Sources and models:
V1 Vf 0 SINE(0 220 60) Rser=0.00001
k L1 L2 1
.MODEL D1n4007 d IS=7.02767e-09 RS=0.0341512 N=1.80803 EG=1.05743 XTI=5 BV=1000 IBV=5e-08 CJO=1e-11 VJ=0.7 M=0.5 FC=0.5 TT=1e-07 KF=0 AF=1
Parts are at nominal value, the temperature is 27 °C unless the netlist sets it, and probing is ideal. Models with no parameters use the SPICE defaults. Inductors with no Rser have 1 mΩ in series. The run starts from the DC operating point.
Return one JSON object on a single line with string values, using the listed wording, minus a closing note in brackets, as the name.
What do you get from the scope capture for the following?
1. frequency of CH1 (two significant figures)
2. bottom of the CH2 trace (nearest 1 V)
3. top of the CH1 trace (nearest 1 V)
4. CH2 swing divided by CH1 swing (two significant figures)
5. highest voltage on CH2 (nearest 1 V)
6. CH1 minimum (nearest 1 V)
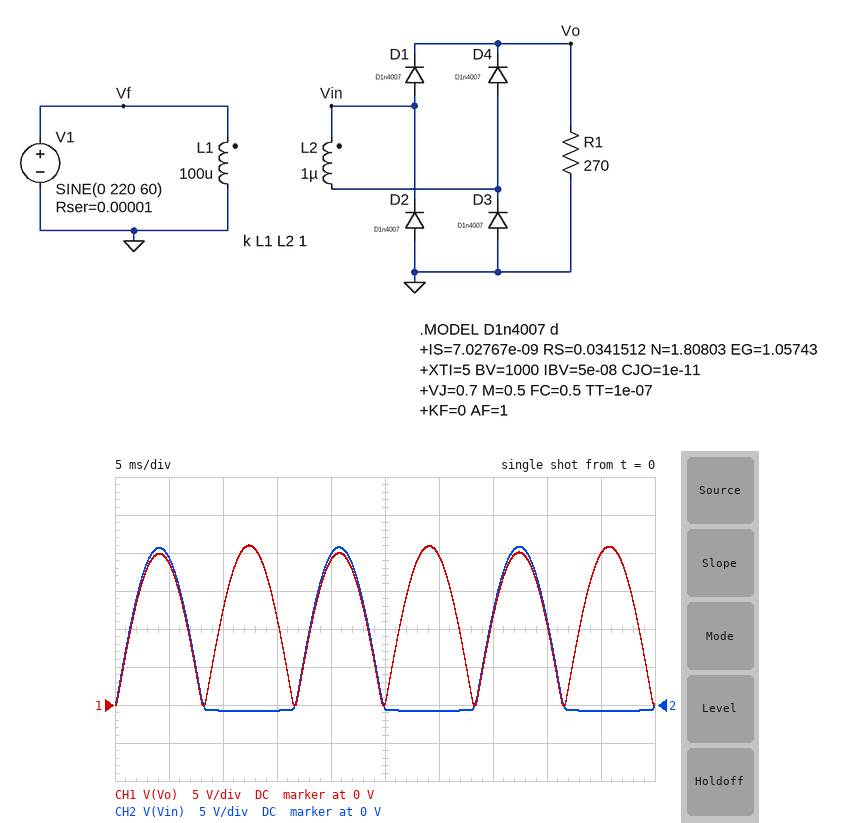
{"frequency of CH1": "120 Hz", "bottom of the CH2 trace": "-1 V", "top of the CH1 trace": "21 V", "CH2 swing divided by CH1 swing": "1.0", "highest voltage on CH2": "21 V", "CH1 minimum": "0 V"}
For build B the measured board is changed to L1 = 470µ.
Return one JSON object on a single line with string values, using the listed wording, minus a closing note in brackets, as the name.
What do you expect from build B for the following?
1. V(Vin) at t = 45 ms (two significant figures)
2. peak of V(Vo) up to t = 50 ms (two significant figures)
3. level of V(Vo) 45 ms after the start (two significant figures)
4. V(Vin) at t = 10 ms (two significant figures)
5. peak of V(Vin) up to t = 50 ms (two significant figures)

{"V(Vin) at t = 45 ms": "-720 mV", "peak of V(Vo) up to t = 50 ms": "8.8 V", "level of V(Vo) 45 ms after the start": "8.3 V", "V(Vin) at t = 10 ms": "-690 mV", "peak of V(Vin) up to t = 50 ms": "9.4 V"}
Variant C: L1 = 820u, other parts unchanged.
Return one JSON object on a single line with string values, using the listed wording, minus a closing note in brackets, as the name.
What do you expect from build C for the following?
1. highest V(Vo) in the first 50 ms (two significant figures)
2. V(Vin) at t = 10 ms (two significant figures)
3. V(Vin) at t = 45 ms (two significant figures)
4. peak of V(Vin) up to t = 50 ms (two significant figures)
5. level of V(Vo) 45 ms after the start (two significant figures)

{"highest V(Vo) in the first 50 ms": "6.3 V", "V(Vin) at t = 10 ms": "-670 mV", "V(Vin) at t = 45 ms": "-700 mV", "peak of V(Vin) up to t = 50 ms": "7.0 V", "level of V(Vo) 45 ms after the start": "5.9 V"}
